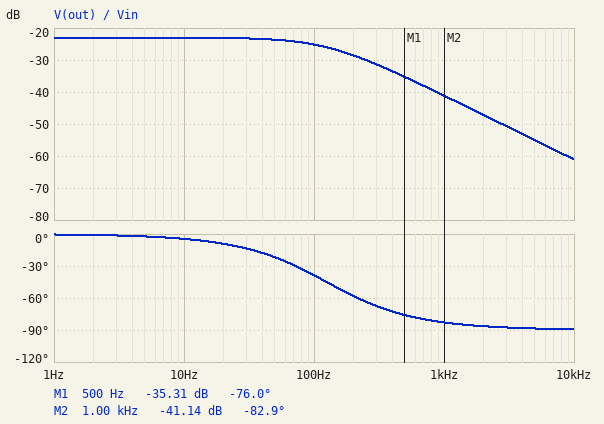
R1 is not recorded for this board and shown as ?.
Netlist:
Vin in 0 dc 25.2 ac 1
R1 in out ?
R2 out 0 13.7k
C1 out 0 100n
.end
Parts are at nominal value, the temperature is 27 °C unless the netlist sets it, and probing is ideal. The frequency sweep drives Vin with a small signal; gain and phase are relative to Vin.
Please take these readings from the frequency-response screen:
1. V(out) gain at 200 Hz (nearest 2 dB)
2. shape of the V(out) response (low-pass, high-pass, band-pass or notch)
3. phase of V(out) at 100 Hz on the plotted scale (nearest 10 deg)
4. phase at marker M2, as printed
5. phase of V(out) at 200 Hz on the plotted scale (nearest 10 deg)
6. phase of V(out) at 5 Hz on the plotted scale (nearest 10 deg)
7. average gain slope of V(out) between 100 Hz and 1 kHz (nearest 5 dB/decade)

-28 dB
low-pass
-40 deg
-82.9 deg
-60 deg
0 deg
-15 dB/decade
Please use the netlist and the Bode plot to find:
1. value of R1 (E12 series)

180 kΩ
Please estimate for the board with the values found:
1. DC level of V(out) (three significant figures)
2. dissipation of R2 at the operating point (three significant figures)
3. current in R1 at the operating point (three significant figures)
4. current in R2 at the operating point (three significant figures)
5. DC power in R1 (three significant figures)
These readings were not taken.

1.78 V
232 µW
130 µA
130 µA
3.05 mW
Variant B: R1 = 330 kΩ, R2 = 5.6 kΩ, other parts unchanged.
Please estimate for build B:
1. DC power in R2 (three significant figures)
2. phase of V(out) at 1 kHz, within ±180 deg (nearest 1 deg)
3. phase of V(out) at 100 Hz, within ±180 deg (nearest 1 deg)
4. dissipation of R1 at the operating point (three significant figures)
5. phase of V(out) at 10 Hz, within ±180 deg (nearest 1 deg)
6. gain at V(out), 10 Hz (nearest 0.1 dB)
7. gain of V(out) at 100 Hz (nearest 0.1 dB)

31.6 µW
-74 deg
-19 deg
1.86 mW
-2 deg
-35.6 dB
-36.0 dB
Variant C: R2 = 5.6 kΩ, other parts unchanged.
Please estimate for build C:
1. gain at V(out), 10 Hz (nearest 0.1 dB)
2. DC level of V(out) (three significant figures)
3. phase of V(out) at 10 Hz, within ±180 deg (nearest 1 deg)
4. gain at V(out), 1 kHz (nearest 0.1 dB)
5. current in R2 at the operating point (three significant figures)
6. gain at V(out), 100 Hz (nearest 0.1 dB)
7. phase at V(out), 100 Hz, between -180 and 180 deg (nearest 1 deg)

-30.4 dB
760 mV
-2 deg
-41.4 dB
136 µA
-30.9 dB
-19 deg
